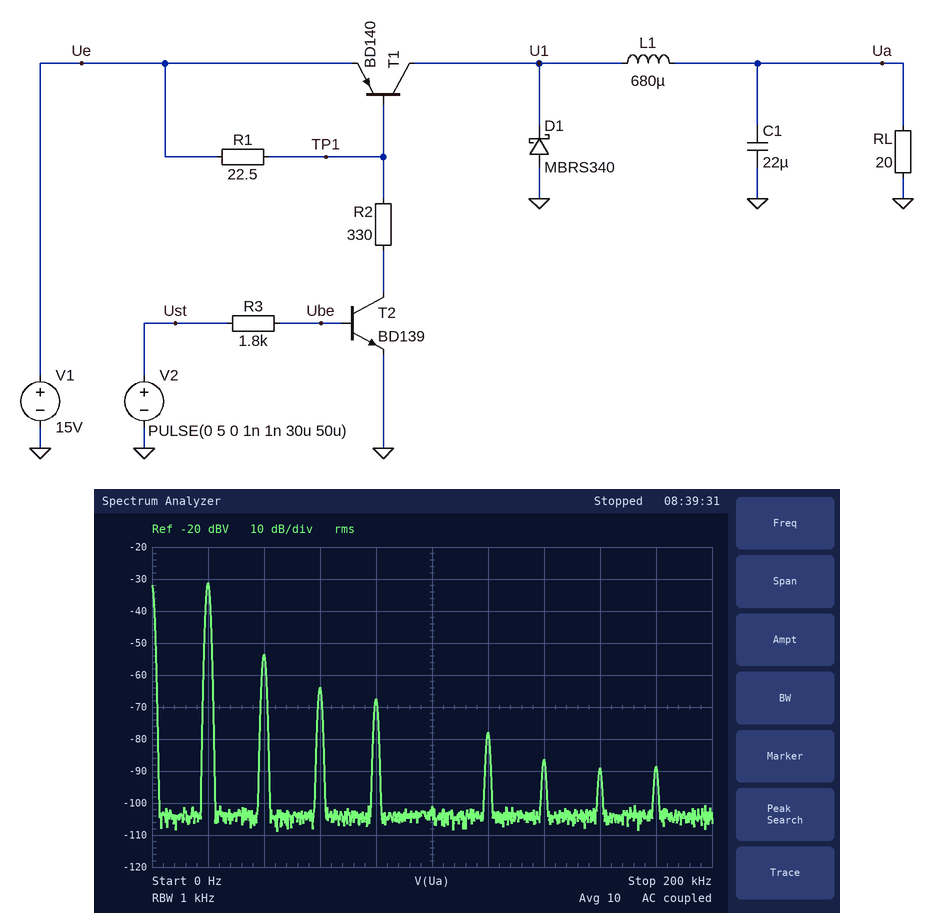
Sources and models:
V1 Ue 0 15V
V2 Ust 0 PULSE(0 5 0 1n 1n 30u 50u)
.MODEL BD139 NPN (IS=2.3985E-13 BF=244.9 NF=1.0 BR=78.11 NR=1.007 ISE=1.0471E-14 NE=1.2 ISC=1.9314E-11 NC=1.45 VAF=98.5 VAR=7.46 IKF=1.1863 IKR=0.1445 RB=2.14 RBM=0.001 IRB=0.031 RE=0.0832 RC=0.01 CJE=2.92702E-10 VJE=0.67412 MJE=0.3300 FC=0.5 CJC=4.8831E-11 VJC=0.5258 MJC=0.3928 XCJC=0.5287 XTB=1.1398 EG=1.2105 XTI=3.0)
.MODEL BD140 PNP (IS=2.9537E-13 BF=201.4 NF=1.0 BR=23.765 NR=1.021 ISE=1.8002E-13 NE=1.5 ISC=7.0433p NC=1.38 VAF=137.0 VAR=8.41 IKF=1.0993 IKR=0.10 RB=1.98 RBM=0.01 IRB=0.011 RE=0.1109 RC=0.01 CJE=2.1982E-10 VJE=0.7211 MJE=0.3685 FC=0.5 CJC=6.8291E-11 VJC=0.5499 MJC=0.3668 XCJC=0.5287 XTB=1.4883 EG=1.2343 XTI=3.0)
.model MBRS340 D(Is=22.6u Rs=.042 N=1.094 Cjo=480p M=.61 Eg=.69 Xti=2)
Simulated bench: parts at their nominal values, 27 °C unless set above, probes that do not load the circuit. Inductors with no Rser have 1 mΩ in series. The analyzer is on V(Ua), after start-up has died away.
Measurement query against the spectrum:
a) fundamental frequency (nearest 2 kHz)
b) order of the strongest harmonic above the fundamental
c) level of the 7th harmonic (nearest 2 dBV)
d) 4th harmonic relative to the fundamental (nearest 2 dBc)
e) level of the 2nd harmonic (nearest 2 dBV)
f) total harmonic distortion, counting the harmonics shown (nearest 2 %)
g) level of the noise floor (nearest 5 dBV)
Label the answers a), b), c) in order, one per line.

a) 20 kHz
b) 2
c) -86 dBV
d) -36 dBc
e) -54 dBV
f) 8 %
g) -105 dBV
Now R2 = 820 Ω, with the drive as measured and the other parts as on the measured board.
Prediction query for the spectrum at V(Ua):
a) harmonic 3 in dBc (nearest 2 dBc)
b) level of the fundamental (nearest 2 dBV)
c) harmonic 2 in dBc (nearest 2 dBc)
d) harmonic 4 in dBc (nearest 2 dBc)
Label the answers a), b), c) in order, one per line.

a) -20 dBc
b) -130 dBV
c) -12 dBc
d) -16 dBc
